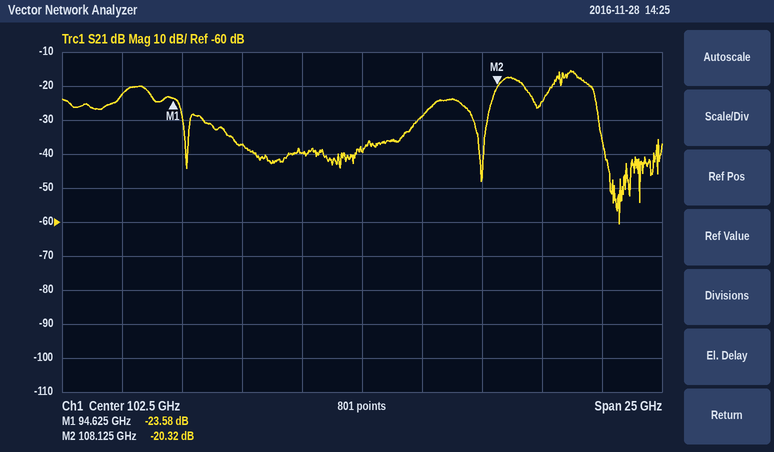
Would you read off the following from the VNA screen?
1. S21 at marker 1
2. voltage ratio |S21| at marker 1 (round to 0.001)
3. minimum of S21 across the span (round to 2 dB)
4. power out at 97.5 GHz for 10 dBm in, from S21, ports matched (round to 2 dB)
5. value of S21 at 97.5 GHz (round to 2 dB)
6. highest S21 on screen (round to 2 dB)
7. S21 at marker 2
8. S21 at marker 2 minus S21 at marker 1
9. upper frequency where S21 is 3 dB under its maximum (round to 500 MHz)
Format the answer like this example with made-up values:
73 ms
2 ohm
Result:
-23.58 dB
0.066
-60 dB
-28 dBm
-38 dB
-16 dB
-20.32 dB
3.26 dB
111.5 GHz
